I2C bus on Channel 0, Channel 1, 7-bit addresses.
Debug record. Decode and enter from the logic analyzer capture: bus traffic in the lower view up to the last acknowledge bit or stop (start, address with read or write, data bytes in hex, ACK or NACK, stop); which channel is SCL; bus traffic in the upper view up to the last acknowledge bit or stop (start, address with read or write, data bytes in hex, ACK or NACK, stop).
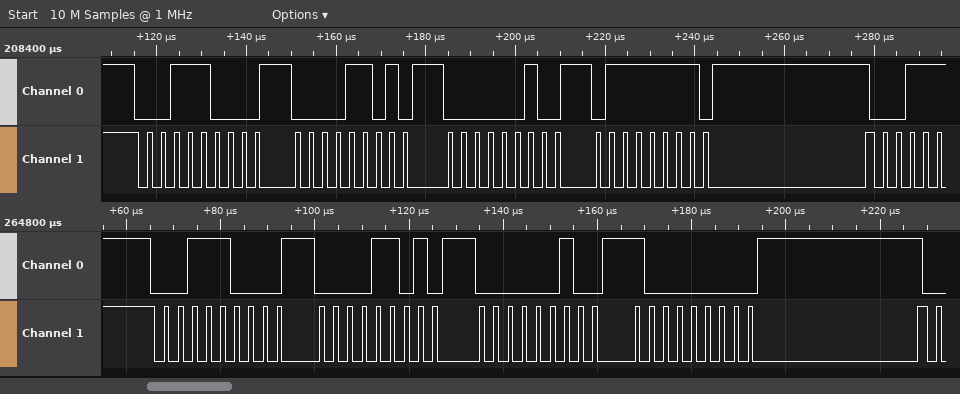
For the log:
start, address 1C write ACK, 0D ACK, 02 ACK, 80 ACK
Channel 1
start, address 1C write ACK, 0D ACK, 02 ACK, 7F ACK
